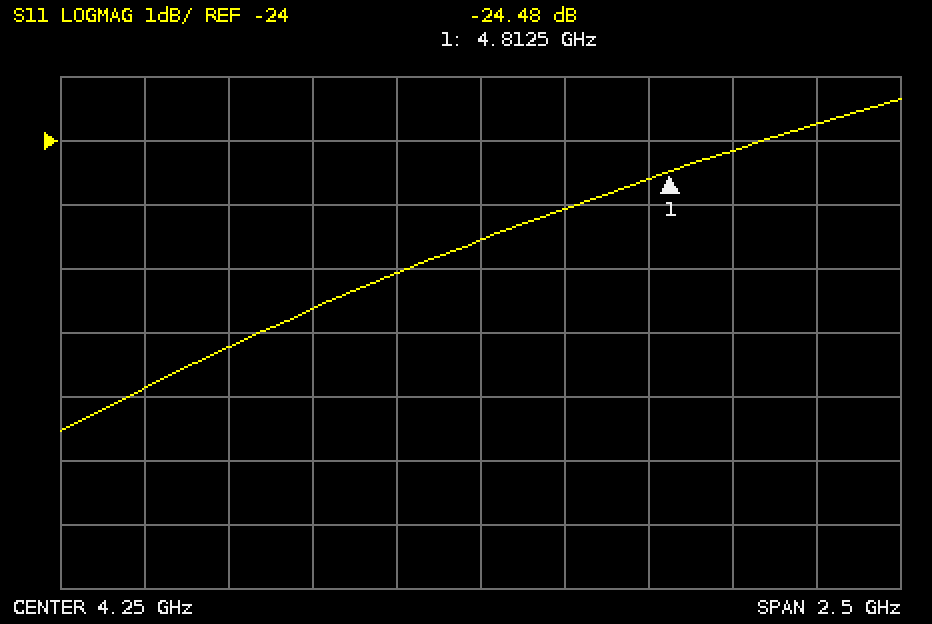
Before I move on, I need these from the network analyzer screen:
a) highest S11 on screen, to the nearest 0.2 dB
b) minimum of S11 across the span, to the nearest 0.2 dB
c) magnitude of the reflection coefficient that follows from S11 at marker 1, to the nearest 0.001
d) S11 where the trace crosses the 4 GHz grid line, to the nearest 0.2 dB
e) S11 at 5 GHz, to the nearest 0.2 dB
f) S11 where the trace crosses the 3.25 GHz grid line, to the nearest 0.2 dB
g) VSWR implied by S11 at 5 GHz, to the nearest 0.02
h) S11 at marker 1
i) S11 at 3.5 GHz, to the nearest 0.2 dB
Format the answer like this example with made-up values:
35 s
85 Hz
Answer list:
-23.4 dB
-28.6 dB
0.060
-26.0 dB
-24.2 dB
-27.8 dB
1.14
-24.48 dB
-27.2 dB
